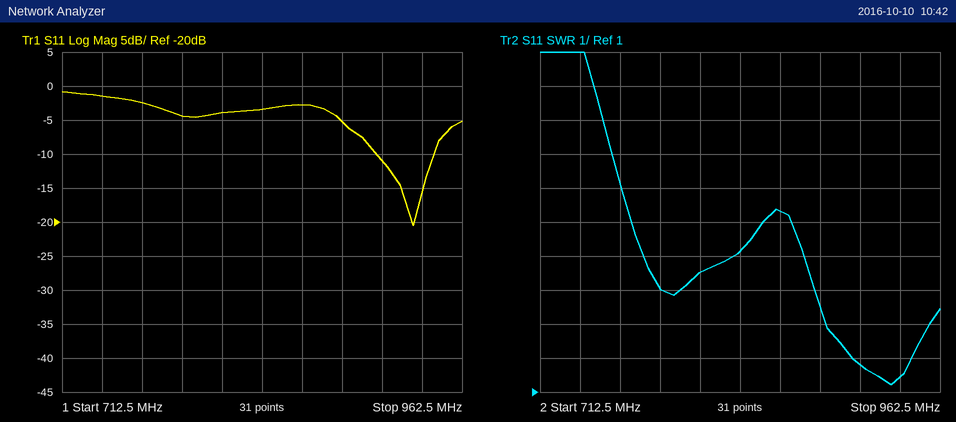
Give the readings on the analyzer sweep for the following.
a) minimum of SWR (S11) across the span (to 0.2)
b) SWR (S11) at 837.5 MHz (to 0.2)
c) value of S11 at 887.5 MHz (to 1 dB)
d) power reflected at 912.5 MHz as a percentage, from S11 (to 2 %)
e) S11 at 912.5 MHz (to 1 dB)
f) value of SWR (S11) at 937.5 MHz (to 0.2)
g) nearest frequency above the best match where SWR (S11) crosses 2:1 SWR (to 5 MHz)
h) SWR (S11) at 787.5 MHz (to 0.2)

1.2
5.2
-5 dB
8 %
-11 dB
1.4
945 MHz
4.0
